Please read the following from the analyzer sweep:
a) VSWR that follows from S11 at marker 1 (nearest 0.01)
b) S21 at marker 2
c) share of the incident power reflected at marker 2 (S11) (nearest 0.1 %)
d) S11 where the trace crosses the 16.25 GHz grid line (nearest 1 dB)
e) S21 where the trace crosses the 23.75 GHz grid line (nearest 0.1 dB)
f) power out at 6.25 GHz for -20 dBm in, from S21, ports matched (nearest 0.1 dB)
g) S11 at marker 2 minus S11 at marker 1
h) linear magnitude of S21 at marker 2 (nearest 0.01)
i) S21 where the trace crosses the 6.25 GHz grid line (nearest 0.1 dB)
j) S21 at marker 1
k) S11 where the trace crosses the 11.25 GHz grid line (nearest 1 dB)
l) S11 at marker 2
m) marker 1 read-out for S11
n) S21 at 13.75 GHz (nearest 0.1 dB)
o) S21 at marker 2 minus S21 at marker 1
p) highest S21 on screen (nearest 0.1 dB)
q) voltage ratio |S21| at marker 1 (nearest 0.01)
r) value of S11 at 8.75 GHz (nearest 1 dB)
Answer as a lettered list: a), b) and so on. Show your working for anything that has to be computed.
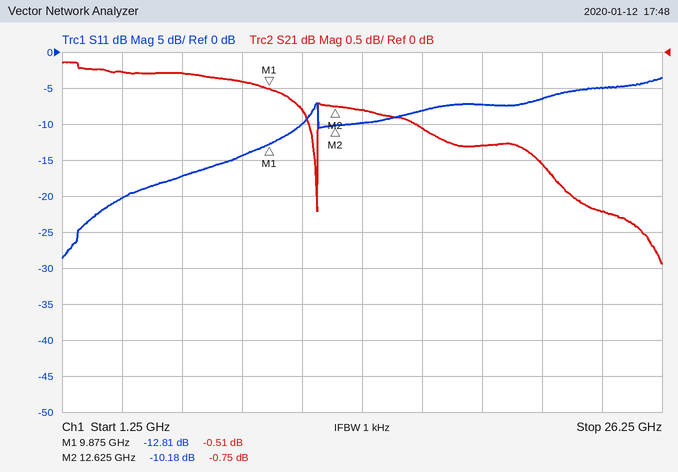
a) (1 + 0.2288)/(1 − 0.2288) ≈ 1.59
b) -0.75 dB
c) 10^(-10.18/10) ≈ 9.6 %
d) -8 dB
e) -2.2 dB
f) -20 dBm + (-0.3 dB) = -20.3 dBm
g) -10.18 − (-12.81) = 2.63 dB
h) 10^(-0.75/20) ≈ 0.92
i) -0.3 dB
j) -0.51 dB
k) -10 dB
l) -10.18 dB
m) -12.81 dB
n) -0.8 dB
o) -0.75 − (-0.51) = -0.24 dB
p) -0.1 dB
q) 10^(-0.51/20) ≈ 0.94
r) -14 dB
